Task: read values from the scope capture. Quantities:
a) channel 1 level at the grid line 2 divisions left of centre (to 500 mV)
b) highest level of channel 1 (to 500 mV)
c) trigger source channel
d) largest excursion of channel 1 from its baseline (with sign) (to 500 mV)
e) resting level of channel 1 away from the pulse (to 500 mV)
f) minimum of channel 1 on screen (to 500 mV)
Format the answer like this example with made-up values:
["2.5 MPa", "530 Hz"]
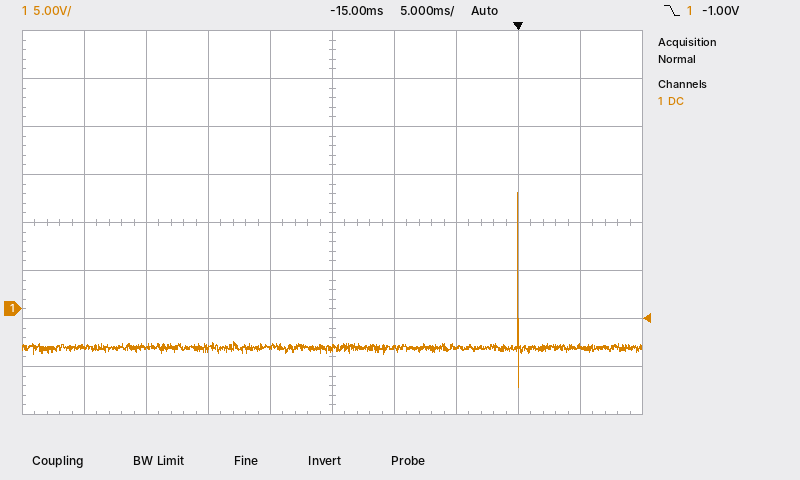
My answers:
["-4.0 V", "12.0 V", "channel 1", "+16.0 V", "-4.0 V", "-8.0 V"]
